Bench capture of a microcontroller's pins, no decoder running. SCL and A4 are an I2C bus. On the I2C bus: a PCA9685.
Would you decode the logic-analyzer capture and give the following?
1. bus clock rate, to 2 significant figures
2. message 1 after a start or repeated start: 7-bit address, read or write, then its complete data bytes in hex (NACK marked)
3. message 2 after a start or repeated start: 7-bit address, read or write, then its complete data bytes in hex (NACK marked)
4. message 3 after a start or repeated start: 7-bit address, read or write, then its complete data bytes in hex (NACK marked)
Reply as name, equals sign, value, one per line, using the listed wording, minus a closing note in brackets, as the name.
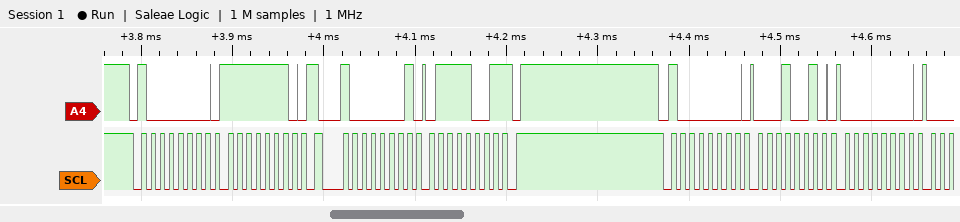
bus clock rate, to 2 significant figures = 100 kHz
message 1 after a start or repeated start: 7-bit address, read or write, then its complete data bytes in hex = 0x40 write: FE
message 2 after a start or repeated start: 7-bit address, read or write, then its complete data bytes in hex = 0x40 read: 79 NACK
message 3 after a start or repeated start: 7-bit address, read or write, then its complete data bytes in hex = 0x40 write: 12 00
